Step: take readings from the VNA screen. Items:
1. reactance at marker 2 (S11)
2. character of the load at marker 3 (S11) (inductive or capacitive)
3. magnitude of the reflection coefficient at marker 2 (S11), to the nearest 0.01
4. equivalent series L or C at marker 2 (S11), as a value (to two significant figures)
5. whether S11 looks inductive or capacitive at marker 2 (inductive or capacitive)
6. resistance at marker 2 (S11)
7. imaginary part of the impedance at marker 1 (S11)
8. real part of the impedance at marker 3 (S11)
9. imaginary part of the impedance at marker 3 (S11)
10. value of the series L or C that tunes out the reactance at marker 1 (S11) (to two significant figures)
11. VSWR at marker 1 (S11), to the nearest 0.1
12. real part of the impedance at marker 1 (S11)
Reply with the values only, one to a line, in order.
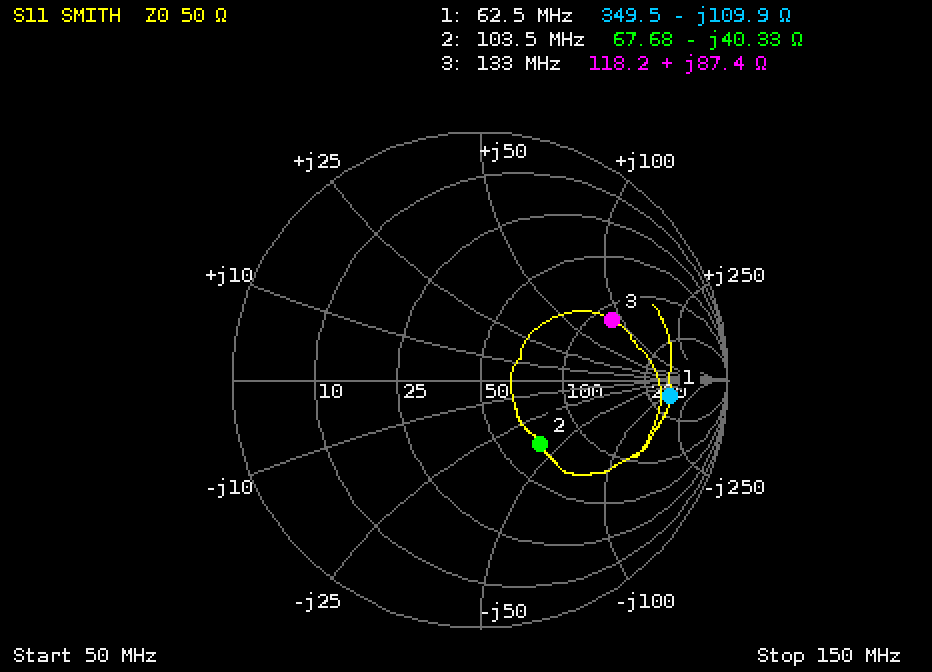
-40.33 Ω
inductive
0.35
38 pF
capacitive
67.68 Ω
-109.9 Ω
118.2 Ω
+87.4 Ω
280 nH
7.7
349.5 Ω
